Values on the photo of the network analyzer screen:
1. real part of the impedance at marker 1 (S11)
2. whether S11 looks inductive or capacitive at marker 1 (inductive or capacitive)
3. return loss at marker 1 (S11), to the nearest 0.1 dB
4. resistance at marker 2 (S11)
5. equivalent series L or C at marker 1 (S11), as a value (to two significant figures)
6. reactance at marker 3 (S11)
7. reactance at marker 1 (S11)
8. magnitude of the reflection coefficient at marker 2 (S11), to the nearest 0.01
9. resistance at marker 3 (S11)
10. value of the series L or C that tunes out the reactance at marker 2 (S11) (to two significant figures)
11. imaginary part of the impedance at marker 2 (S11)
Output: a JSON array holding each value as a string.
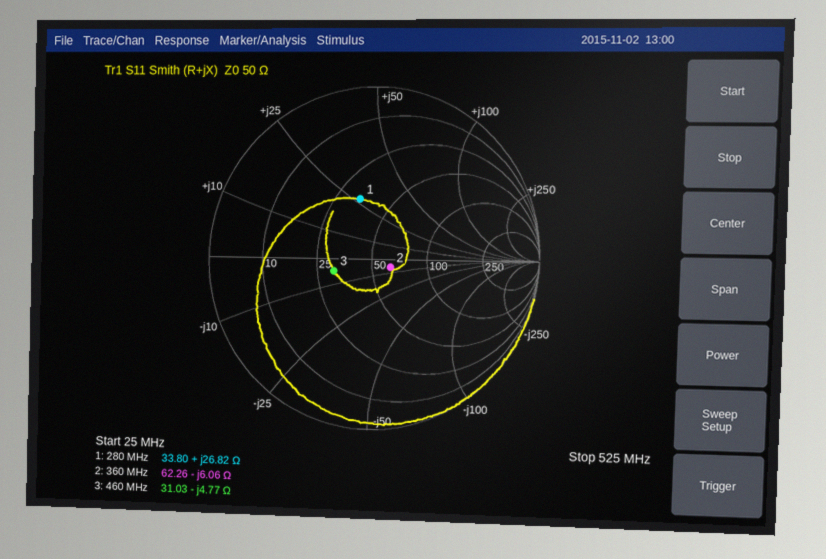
["33.80 Ω", "inductive", "9.0 dB", "62.26 Ω", "15 nH", "-4.77 Ω", "+26.82 Ω", "0.12", "31.03 Ω", "2.7 nH", "-6.06 Ω"]
